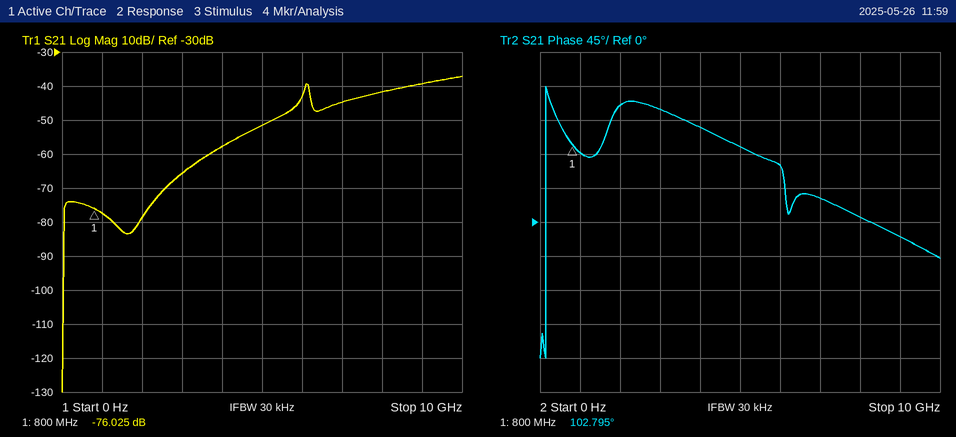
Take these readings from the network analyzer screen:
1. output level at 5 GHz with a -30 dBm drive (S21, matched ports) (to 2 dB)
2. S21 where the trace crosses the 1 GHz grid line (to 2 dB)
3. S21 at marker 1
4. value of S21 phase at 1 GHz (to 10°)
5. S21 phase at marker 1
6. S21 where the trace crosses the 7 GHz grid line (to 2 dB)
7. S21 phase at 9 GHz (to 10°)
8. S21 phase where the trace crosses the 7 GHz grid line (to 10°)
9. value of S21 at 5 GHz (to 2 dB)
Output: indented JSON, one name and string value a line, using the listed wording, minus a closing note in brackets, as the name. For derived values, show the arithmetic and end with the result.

{
  "output level at 5 GHz with a -30 dBm drive (S21, matched ports)": "-30 dBm + (-52 dB) = -82 dBm",
  "S21 where the trace crosses the 1 GHz grid line": "-78 dB",
  "S21 at marker 1": "-76.025 dB",
  "value of S21 phase at 1 GHz": "90°",
  "S21 phase at marker 1": "102.795°",
  "S21 where the trace crosses the 7 GHz grid line": "-44 dB",
  "S21 phase at 9 GHz": "-20°",
  "S21 phase where the trace crosses the 7 GHz grid line": "30°",
  "value of S21 at 5 GHz": "-52 dB"
}
